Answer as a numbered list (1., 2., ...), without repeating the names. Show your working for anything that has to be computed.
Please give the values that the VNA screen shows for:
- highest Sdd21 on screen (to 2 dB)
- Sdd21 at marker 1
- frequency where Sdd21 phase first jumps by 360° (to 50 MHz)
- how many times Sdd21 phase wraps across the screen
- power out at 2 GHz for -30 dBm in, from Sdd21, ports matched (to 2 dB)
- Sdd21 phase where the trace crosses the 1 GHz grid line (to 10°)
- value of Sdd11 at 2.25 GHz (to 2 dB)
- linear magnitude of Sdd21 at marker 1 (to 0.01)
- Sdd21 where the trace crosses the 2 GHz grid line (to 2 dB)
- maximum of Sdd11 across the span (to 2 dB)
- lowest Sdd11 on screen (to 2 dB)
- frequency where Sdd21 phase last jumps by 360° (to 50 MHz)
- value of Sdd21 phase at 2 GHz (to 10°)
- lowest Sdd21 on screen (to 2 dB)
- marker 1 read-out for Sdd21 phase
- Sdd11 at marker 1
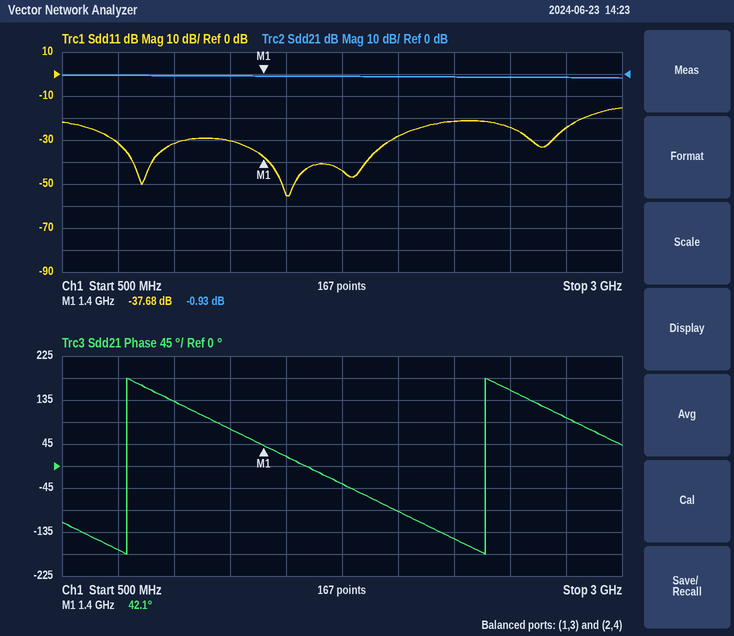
1. 0 dB
2. -0.93 dB
3. 800 MHz
4. 2
5. -30 dBm + (-2 dB) = -32 dBm
6. 130°
7. -22 dB
8. 10^(-0.93/20) ≈ 0.90
9. -2 dB
10. -16 dB
11. -56 dB
12. 2.40 GHz
13. -90°
14. -2 dB
15. 42.1°
16. -37.68 dB
